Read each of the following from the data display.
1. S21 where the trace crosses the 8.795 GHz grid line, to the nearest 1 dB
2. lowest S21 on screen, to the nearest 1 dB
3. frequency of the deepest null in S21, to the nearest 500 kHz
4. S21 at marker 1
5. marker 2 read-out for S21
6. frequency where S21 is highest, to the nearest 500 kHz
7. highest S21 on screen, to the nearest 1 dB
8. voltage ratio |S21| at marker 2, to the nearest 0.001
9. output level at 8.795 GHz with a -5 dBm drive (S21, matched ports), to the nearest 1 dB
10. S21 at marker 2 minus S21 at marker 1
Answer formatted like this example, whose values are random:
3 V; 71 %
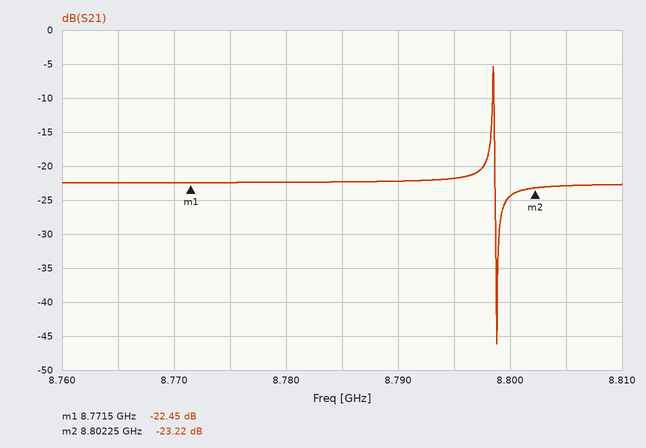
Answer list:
-22 dB; -46 dB; 8.7990 GHz; -22.45 dB; -23.22 dB; 8.7985 GHz; -5 dB; 0.069; -27 dBm; -0.77 dB
